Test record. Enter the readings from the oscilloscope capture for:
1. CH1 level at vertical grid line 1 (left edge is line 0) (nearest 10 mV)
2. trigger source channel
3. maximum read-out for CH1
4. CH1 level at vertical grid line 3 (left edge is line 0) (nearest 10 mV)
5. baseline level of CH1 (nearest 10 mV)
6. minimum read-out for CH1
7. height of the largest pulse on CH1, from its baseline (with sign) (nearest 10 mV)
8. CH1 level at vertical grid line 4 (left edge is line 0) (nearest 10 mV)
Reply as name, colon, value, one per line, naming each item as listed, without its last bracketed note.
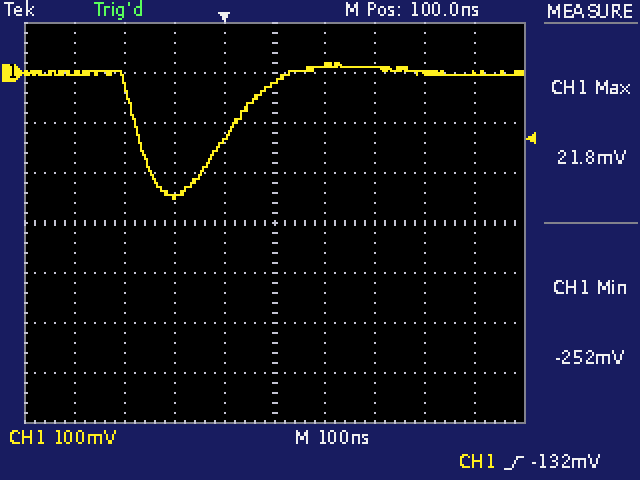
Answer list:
CH1 level at vertical grid line 1 (left edge is line 0): 0 mV
trigger source channel: CH1
maximum read-out for CH1: 21.8 mV
CH1 level at vertical grid line 3 (left edge is line 0): -250 mV
baseline level of CH1: 0 mV
minimum read-out for CH1: -252 mV
height of the largest pulse on CH1, from its baseline (with sign): -250 mV
CH1 level at vertical grid line 4 (left edge is line 0): -130 mV
